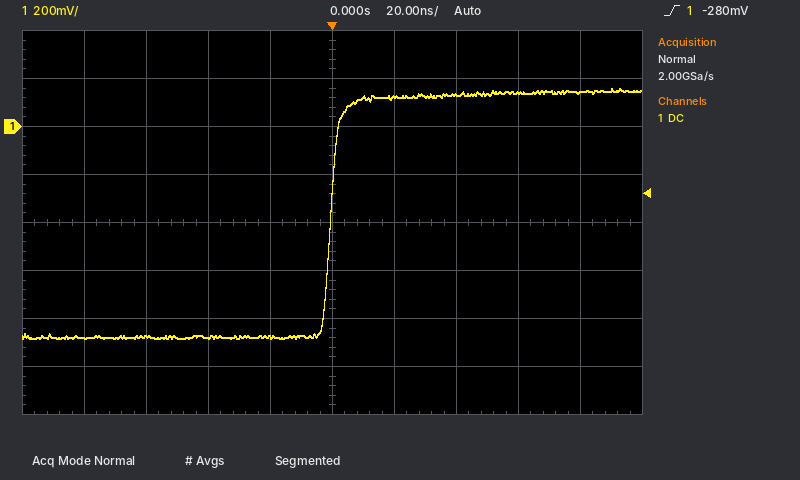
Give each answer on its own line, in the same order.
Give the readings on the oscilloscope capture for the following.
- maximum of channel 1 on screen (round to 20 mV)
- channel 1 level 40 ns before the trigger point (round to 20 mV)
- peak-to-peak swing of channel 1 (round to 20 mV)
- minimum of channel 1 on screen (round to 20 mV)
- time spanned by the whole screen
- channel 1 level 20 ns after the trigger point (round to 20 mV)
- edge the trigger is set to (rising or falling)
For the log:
160 mV
-880 mV
1.04 V
-880 mV
200 ns
120 mV
rising
